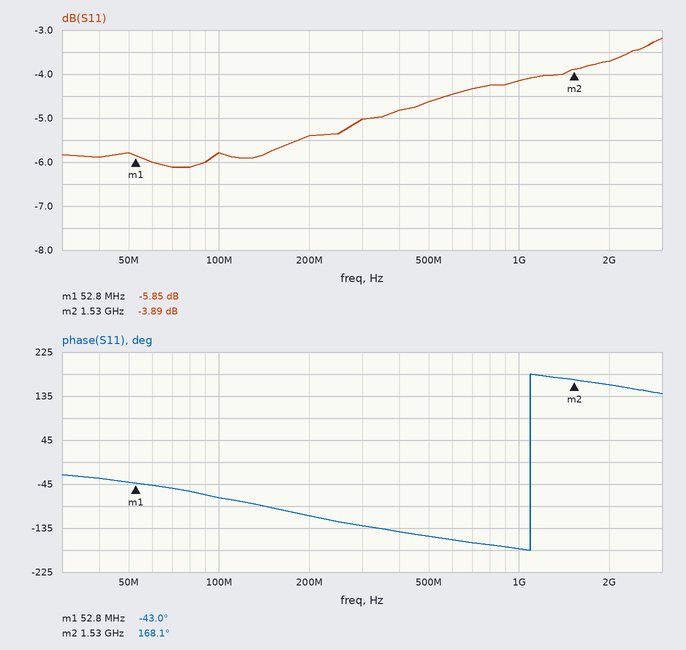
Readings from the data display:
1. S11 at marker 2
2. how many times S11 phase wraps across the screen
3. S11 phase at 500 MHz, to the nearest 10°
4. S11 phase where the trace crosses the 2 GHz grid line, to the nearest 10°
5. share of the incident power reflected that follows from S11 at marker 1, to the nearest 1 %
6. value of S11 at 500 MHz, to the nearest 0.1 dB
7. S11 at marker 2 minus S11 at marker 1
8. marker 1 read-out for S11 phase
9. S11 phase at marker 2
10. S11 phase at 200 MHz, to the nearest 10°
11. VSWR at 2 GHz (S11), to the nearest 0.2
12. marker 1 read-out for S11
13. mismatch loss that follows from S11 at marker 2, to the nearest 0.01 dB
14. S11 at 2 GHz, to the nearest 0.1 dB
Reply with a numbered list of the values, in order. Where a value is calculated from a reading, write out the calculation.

1. -3.89 dB
2. 1
3. -150°
4. 160°
5. 10^(-5.85/10) ≈ 26 %
6. -4.6 dB
7. -3.89 − (-5.85) = 1.96 dB
8. -43.0°
9. 168.1°
10. -110°
11. |Γ| = 10^(-3.7/20) = 0.6531; VSWR = (1 + 0.6531)/(1 − 0.6531) ≈ 4.8
12. -5.85 dB
13. −10 log10(1 − 10^(-3.89/10)) ≈ 2.28 dB
14. -3.7 dB
